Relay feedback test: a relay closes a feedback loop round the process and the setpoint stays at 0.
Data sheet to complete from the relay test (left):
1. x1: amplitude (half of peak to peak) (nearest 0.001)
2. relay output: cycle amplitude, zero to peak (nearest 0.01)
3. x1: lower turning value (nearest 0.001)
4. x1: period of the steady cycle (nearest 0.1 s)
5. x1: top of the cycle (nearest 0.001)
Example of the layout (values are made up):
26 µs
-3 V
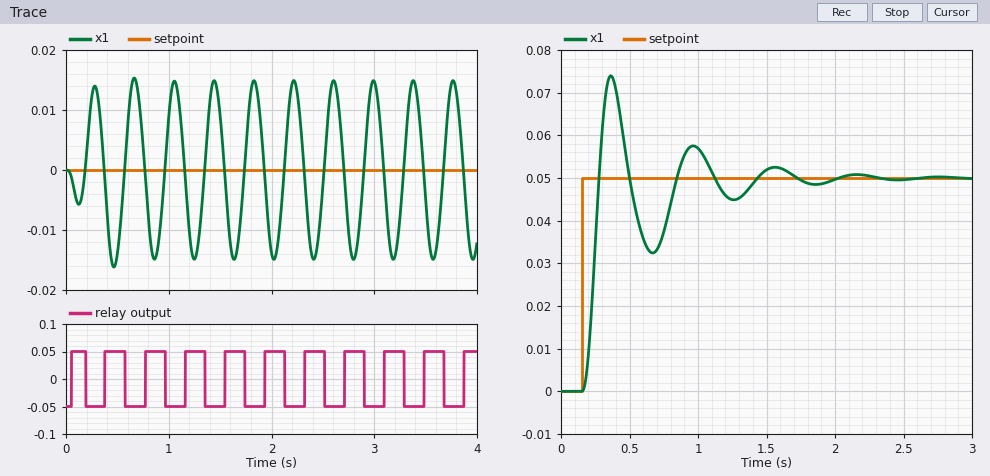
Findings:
0.015
0.05
-0.015
0.4 s
0.015
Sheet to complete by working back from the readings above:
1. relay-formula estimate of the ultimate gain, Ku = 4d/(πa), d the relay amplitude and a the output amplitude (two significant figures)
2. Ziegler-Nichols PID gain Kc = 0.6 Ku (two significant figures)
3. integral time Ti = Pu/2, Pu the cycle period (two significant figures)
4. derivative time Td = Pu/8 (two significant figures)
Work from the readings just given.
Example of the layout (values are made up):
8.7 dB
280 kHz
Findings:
4.2
2.5
0.20 s
0.050 s
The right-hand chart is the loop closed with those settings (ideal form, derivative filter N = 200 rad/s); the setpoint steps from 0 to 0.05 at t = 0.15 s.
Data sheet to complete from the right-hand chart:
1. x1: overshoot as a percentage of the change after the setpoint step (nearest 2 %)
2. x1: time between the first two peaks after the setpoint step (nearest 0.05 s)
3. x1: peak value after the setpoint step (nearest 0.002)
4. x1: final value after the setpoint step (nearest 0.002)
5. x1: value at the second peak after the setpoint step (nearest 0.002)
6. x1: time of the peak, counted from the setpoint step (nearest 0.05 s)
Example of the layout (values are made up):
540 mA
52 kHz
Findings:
48 %
0.60 s
0.074
0.050
0.058
0.20 s
